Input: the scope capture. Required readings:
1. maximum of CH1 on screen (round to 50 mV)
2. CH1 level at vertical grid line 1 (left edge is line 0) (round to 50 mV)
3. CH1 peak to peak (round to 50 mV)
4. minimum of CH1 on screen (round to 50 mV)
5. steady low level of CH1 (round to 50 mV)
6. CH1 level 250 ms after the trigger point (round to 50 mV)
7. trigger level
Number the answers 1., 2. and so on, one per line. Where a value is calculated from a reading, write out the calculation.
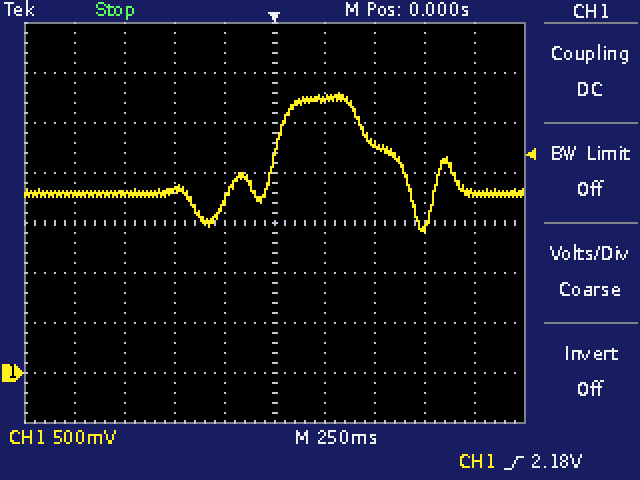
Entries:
1. 2.80 V
2. 1.80 V
3. 2.80 V − (1.40 V) = 1.40 V
4. 1.40 V
5. 1.80 V
6. 2.75 V
7. 2.18 V
